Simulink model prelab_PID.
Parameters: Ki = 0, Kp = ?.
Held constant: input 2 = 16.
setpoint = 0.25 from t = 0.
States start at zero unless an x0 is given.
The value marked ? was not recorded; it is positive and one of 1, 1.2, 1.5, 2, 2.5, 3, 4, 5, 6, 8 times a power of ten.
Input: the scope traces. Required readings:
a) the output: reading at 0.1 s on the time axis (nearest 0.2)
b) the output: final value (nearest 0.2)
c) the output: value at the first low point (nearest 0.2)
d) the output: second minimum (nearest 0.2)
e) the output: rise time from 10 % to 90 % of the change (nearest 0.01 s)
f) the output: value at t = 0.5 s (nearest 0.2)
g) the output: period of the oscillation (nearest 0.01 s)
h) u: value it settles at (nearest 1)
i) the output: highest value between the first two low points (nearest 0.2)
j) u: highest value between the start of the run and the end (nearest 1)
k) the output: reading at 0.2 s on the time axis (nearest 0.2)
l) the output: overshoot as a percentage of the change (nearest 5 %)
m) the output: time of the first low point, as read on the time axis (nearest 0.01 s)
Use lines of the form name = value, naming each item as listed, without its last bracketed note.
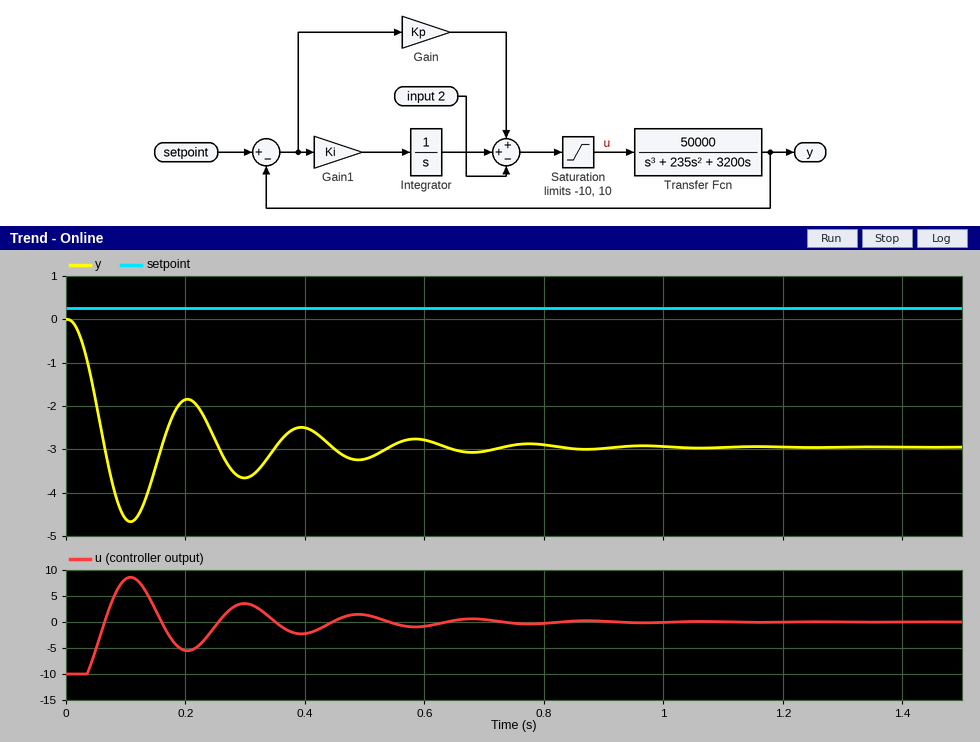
the output: reading at 0.1 s on the time axis = -4.6
the output: final value = -3.0
the output: value at the first low point = -4.6
the output: second minimum = -3.6
the output: rise time from 10 % to 90 % of the change = 0.04 s
the output: value at t = 0.5 s = -3.2
the output: period of the oscillation = 0.19 s
u: value it settles at = 0
the output: highest value between the first two low points = -1.8
u: highest value between the start of the run and the end = 9
the output: reading at 0.2 s on the time axis = -1.8
the output: overshoot as a percentage of the change = 60 %
the output: time of the first low point, as read on the time axis = 0.11 s
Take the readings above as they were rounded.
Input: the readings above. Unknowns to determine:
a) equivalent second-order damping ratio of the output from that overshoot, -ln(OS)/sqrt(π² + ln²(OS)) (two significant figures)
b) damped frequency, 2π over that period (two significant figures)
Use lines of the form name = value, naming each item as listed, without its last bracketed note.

equivalent second-order damping ratio of the output from that overshoot, -ln(OS)/sqrt(π² + ln²(OS)) = 0.16
damped frequency, 2π over that period = 33 rad/s
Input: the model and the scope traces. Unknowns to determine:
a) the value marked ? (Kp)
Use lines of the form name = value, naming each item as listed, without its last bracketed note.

the value marked ? = 5
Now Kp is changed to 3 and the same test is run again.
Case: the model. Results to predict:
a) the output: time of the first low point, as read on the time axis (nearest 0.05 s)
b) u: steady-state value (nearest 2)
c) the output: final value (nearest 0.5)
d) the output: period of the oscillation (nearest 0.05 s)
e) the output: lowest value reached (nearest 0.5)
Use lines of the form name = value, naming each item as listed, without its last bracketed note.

the output: time of the first low point, as read on the time axis = 0.15 s
u: steady-state value = 0
the output: final value = -5.0
the output: period of the oscillation = 0.25 s
the output: lowest value reached = -7.5
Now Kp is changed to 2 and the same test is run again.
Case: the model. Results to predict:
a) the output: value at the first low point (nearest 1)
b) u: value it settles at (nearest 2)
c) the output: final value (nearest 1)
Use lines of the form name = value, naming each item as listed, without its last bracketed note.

the output: value at the first low point = -10
u: value it settles at = 0
the output: final value = -8
